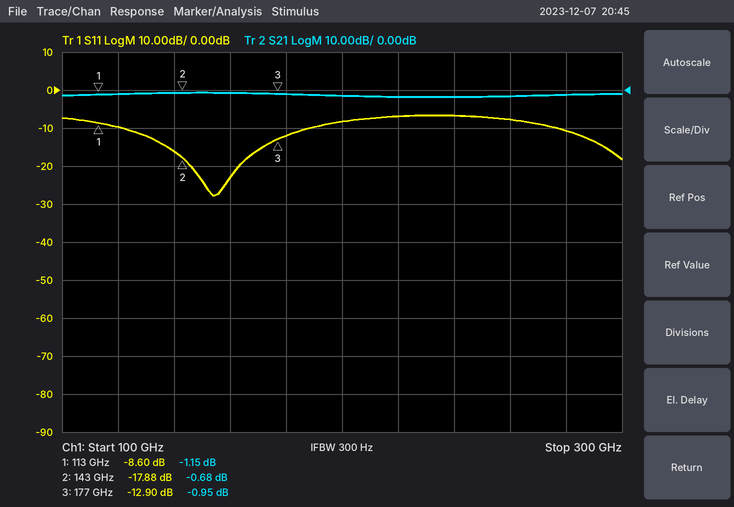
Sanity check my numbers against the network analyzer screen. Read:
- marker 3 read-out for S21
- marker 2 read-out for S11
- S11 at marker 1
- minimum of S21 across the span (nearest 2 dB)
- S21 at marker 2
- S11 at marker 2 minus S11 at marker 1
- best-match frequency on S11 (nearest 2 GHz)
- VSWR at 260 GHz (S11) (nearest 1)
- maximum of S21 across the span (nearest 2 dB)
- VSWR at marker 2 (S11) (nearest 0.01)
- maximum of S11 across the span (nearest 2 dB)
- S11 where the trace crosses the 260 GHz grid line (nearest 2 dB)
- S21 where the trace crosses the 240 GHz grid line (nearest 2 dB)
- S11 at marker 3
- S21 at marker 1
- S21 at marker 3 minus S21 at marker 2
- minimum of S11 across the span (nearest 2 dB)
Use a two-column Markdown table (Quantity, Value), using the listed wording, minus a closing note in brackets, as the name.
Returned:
| Quantity | Value |
|---|---|
| marker 3 read-out for S21 | -0.95 dB |
| marker 2 read-out for S11 | -17.88 dB |
| S11 at marker 1 | -8.60 dB |
| minimum of S21 across the span | -2 dB |
| S21 at marker 2 | -0.68 dB |
| S11 at marker 2 minus S11 at marker 1 | -9.28 dB |
| best-match frequency on S11 | 154 GHz |
| VSWR at 260 GHz (S11) | 2 |
| maximum of S21 across the span | 0 dB |
| VSWR at marker 2 (S11) | 1.29 |
| maximum of S11 across the span | -6 dB |
| S11 where the trace crosses the 260 GHz grid line | -8 dB |
| S21 where the trace crosses the 240 GHz grid line | -2 dB |
| S11 at marker 3 | -12.90 dB |
| S21 at marker 1 | -1.15 dB |
| S21 at marker 3 minus S21 at marker 2 | -0.27 dB |
| minimum of S11 across the span | -28 dB |
